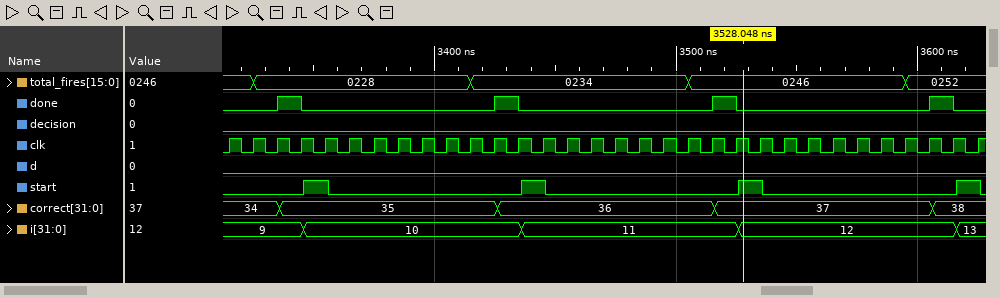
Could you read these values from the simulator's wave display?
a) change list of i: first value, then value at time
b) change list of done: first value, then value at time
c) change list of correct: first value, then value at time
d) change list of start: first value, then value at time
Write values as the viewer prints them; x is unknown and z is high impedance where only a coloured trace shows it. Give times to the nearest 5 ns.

9, 10 at 3345 ns, 11 at 3435 ns, 12 at 3525 ns, 13 at 3615 ns
0, 1 at 3335 ns, 0 at 3345 ns, 1 at 3425 ns, 0 at 3435 ns, 1 at 3515 ns, 0 at 3525 ns, 1 at 3605 ns, 0 at 3615 ns
34, 35 at 3335 ns, 36 at 3425 ns, 37 at 3515 ns, 38 at 3605 ns
0, 1 at 3345 ns, 0 at 3355 ns, 1 at 3435 ns, 0 at 3445 ns, 1 at 3525 ns, 0 at 3535 ns, 1 at 3615 ns, 0 at 3625 ns
